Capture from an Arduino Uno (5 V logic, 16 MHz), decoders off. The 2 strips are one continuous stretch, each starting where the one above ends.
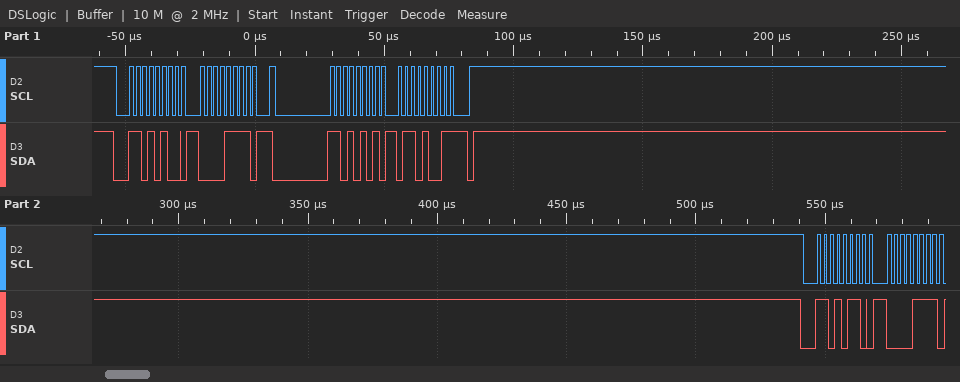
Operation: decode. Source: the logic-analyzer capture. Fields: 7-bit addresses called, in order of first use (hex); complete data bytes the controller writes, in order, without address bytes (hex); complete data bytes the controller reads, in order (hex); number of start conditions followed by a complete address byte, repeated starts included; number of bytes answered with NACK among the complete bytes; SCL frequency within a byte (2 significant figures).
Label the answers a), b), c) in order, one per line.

a) 0x6A 0x6B
b) 0F 0F
c) 69
d) 3
e) 1
f) 400 kHz
